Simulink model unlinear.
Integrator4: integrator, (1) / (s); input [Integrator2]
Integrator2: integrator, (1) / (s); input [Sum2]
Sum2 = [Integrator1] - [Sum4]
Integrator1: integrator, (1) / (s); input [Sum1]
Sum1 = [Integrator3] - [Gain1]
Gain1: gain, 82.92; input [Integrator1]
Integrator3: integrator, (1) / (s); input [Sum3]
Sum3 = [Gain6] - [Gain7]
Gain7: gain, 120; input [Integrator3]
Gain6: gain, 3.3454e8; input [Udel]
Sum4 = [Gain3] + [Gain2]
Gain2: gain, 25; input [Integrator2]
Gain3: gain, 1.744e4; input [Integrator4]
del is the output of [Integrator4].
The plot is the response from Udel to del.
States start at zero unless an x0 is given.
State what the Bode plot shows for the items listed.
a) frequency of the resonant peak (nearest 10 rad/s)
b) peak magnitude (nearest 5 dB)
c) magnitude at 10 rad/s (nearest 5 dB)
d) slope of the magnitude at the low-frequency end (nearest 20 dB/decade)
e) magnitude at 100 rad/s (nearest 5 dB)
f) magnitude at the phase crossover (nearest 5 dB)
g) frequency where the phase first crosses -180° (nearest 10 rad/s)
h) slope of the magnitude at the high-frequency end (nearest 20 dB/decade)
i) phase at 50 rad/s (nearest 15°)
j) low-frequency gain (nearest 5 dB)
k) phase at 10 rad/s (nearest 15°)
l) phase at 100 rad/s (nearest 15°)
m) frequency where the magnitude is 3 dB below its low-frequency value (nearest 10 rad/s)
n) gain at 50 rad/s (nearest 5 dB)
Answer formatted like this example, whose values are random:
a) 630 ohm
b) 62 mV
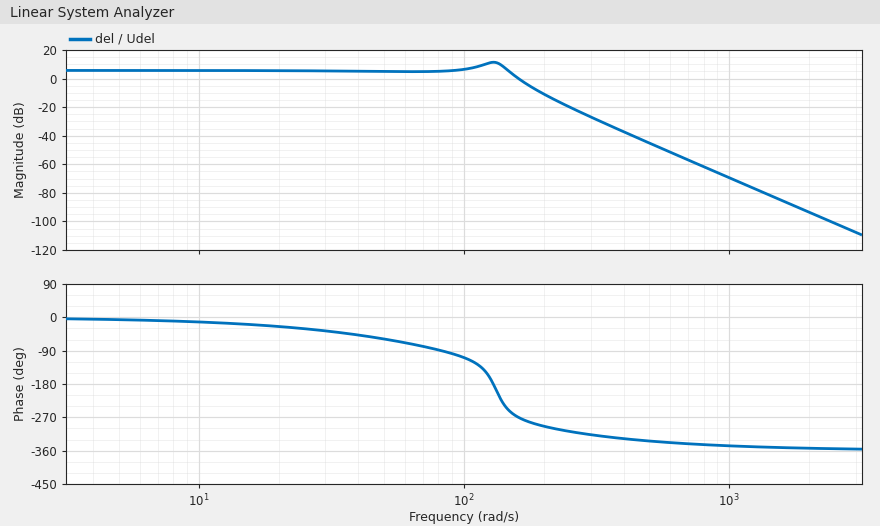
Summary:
a) 130 rad/s
b) 10 dB
c) 5 dB
d) 0 dB/decade
e) 5 dB
f) 10 dB
g) 130 rad/s
h) -80 dB/decade
i) -60°
j) 5 dB
k) -15°
l) -105°
m) 150 rad/s
n) 5 dB
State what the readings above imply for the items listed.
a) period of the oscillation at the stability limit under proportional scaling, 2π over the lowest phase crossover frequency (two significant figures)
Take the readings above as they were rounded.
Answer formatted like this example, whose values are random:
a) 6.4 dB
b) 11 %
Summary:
a) 0.048 s
